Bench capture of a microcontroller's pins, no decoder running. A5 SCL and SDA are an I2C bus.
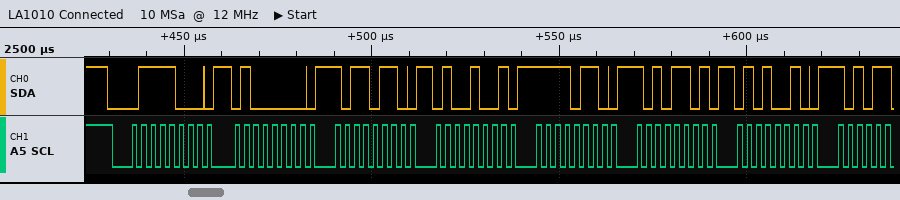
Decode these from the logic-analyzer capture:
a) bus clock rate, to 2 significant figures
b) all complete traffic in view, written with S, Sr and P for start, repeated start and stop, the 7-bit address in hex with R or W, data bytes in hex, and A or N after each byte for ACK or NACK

400 kHz
S 3CW A 40 A B6 A 49 A F6 A AD A 52 A
